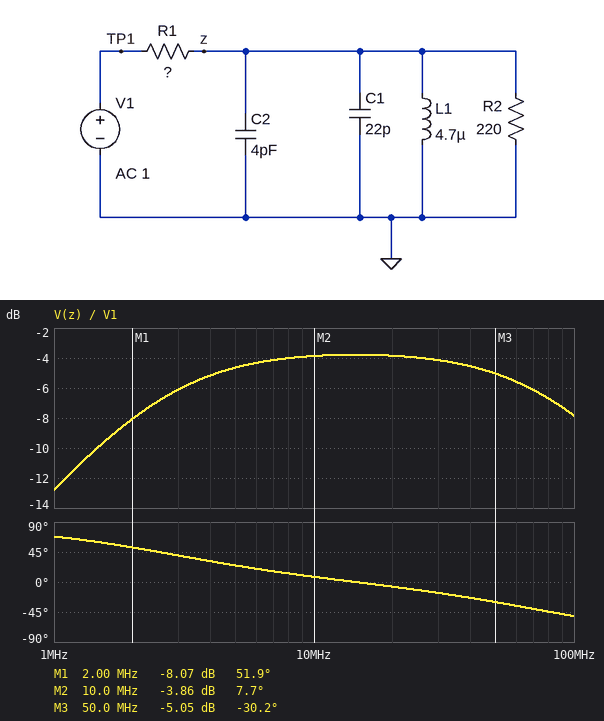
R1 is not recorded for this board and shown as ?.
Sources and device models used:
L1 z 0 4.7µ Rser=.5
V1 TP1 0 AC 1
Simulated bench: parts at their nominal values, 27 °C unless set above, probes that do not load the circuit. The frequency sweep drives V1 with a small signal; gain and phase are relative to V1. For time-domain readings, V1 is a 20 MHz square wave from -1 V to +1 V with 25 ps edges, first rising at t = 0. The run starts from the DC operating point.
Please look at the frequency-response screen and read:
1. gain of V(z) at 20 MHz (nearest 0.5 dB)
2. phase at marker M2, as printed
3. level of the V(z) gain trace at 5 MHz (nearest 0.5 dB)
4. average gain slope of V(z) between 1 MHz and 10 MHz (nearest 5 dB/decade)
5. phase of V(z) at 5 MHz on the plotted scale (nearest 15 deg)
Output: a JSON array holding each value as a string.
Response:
["-4.0 dB", "7.7 deg", "-4.5 dB", "10 dB/decade", "30 deg"]
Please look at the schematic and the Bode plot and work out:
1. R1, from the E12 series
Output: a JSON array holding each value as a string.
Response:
["120 Ω"]
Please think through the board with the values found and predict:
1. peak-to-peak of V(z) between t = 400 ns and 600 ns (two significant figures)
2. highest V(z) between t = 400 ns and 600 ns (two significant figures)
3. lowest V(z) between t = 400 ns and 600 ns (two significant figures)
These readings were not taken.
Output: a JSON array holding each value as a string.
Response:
["1.4 V", "700 mV", "-700 mV"]
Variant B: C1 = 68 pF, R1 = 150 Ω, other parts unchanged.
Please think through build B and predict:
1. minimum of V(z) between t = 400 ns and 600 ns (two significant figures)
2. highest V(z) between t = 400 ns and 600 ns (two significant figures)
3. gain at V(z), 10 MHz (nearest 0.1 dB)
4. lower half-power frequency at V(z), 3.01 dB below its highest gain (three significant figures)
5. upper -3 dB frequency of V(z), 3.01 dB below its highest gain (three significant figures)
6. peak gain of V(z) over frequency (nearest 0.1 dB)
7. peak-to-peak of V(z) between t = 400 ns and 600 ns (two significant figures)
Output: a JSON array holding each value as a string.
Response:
["-570 mV", "570 mV", "-4.6 dB", "2.73 MHz", "27.5 MHz", "-4.5 dB", "1.1 V"]
